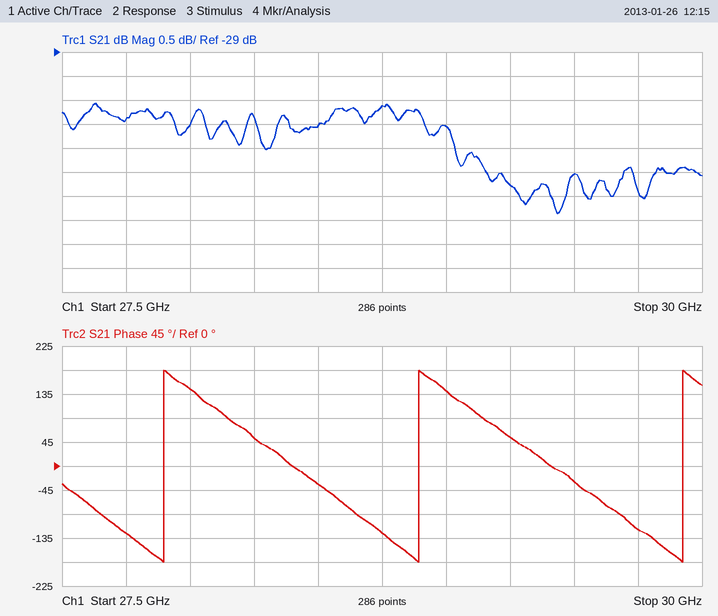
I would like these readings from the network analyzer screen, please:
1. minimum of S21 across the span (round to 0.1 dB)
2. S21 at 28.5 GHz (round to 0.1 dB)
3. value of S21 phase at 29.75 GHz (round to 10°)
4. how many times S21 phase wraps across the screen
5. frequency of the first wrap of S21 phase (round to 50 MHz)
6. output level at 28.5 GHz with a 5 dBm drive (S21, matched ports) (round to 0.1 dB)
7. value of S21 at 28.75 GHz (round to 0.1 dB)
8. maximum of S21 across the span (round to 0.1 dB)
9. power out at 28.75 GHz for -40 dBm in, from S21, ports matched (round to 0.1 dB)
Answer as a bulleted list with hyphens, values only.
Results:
- -32.4 dB
- -30.5 dB
- -120°
- 3
- 27.90 GHz
- -25.5 dBm
- -30.1 dB
- -30.1 dB
- -70.1 dBm
